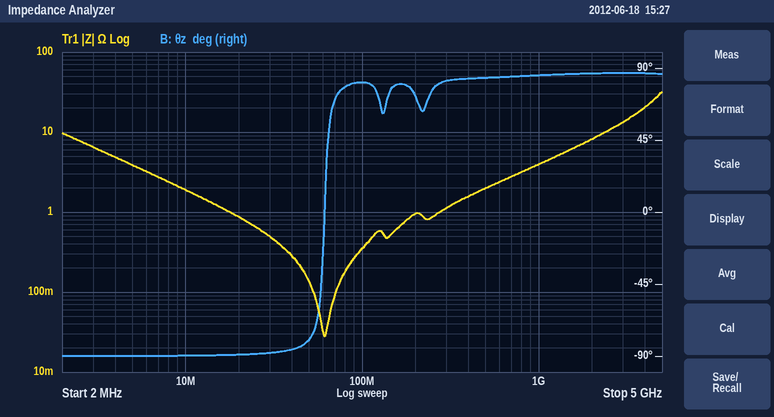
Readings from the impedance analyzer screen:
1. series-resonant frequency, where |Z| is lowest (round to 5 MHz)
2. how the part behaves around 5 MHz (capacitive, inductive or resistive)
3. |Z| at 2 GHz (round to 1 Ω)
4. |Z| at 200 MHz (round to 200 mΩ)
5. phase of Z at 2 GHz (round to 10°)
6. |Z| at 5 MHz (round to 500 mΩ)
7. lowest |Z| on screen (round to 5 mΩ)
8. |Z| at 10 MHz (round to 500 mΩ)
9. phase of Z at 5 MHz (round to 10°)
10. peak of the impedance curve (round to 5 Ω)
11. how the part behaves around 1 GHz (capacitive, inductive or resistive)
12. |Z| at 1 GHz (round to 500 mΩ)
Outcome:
60 MHz
capacitive
8 Ω
1.0 Ω
90°
4.0 Ω
30 mΩ
2.0 Ω
-90°
30 Ω
inductive
4.0 Ω
